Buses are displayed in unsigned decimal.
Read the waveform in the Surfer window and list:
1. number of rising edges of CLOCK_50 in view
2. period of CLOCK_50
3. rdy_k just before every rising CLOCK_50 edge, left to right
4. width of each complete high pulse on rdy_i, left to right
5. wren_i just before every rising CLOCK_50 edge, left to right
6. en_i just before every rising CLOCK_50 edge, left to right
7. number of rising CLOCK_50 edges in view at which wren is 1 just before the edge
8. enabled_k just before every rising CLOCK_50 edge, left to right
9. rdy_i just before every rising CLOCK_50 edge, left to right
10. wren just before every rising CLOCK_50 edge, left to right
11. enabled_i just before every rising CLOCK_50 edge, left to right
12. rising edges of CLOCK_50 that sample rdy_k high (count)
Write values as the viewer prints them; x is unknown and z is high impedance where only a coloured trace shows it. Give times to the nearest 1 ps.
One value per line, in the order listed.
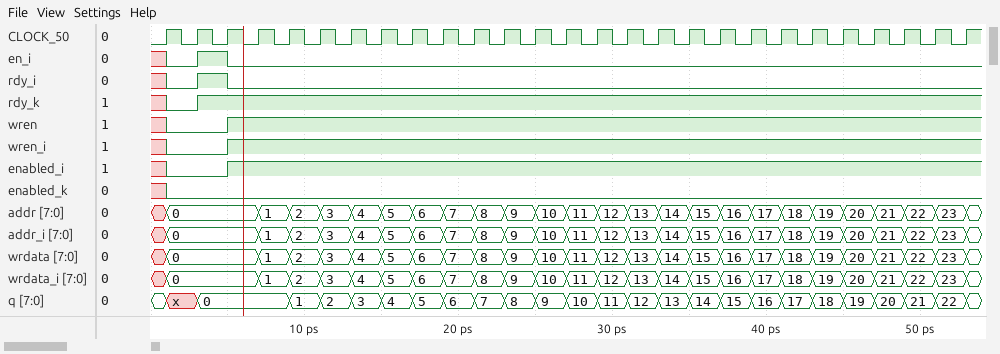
27
2 ps
x 0 1 1 1 1 1 1 1 1 1 1 1 1 1 1 1 1 1 1 1 1 1 1 1 1 1
2 ps
x 0 0 1 1 1 1 1 1 1 1 1 1 1 1 1 1 1 1 1 1 1 1 1 1 1 1
x 0 1 0 0 0 0 0 0 0 0 0 0 0 0 0 0 0 0 0 0 0 0 0 0 0 0
24
x 0 0 0 0 0 0 0 0 0 0 0 0 0 0 0 0 0 0 0 0 0 0 0 0 0 0
x 0 1 0 0 0 0 0 0 0 0 0 0 0 0 0 0 0 0 0 0 0 0 0 0 0 0
x 0 0 1 1 1 1 1 1 1 1 1 1 1 1 1 1 1 1 1 1 1 1 1 1 1 1
x 0 0 1 1 1 1 1 1 1 1 1 1 1 1 1 1 1 1 1 1 1 1 1 1 1 1
25
